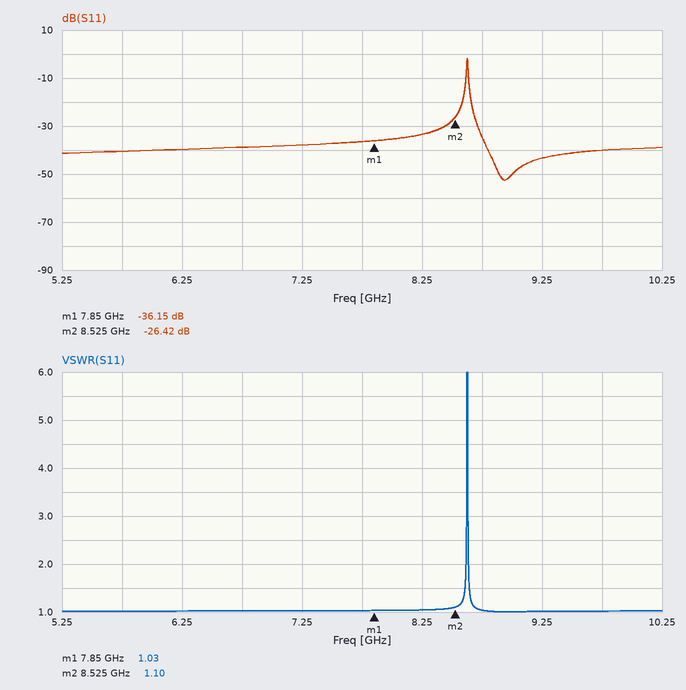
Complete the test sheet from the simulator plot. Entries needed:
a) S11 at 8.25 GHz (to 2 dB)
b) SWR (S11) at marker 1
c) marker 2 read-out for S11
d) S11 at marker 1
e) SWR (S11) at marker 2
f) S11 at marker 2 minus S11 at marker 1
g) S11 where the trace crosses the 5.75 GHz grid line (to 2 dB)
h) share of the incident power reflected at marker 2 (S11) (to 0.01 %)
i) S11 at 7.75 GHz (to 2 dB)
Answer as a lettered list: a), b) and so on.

a) -34 dB
b) 1.03
c) -26.42 dB
d) -36.15 dB
e) 1.10
f) 9.73 dB
g) -40 dB
h) 0.23 %
i) -36 dB
